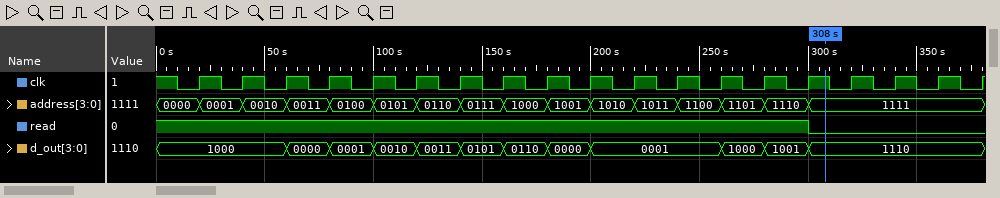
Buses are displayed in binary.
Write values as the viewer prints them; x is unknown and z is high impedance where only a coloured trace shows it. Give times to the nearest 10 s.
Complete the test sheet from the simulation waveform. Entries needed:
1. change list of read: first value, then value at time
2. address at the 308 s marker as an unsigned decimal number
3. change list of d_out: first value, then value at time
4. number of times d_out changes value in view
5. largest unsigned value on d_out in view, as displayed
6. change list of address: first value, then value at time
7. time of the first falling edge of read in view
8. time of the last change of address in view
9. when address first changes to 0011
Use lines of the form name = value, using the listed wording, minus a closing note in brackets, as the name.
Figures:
change list of read: first value, then value at time = 1, 0 at 300 s
address at the 308 s marker as an unsigned decimal number = 15
change list of d_out: first value, then value at time = 1000, 0000 at 60 s, 0001 at 80 s, 0010 at 100 s, 0011 at 120 s, 0101 at 140 s, 0110 at 160 s, 0000 at 180 s, 0001 at 200 s, 1000 at 260 s, 1001 at 280 s, 1110 at 300 s
number of times d_out changes value in view = 11
largest unsigned value on d_out in view, as displayed = 1110
change list of address: first value, then value at time = 0000, 0001 at 20 s, 0010 at 40 s, 0011 at 60 s, 0100 at 80 s, 0101 at 100 s, 0110 at 120 s, 0111 at 140 s, 1000 at 160 s, 1001 at 180 s, 1010 at 200 s, 1011 at 220 s, 1100 at 240 s, 1101 at 260 s, 1110 at 280 s, 1111 at 300 s
time of the first falling edge of read in view = 300 s
time of the last change of address in view = 300 s
when address first changes to 0011 = 60 s
